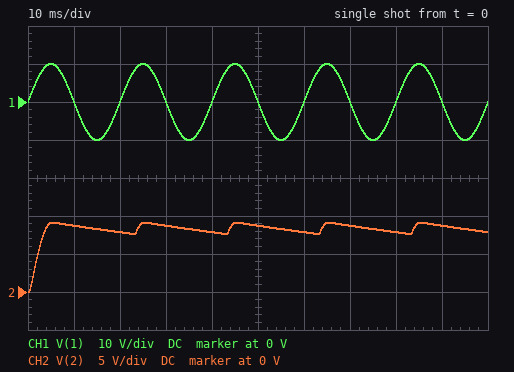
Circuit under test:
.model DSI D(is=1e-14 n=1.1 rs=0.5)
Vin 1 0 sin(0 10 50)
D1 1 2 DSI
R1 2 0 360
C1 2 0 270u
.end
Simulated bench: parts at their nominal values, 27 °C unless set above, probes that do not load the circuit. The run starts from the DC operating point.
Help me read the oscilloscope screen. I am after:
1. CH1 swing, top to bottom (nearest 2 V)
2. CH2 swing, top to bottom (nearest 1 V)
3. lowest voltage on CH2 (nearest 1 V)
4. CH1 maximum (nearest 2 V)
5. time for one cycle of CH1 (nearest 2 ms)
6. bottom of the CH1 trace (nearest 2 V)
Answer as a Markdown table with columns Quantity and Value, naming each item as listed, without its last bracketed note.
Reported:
| Quantity | Value |
|---|---|
| CH1 swing, top to bottom | 20 V |
| CH2 swing, top to bottom | 9 V |
| lowest voltage on CH2 | 0 V |
| CH1 maximum | 10 V |
| time for one cycle of CH1 | 20 ms |
| bottom of the CH1 trace | -10 V |
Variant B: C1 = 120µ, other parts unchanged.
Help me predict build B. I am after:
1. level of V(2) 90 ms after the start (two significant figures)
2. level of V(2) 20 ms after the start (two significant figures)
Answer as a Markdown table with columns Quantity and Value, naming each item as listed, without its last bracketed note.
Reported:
| Quantity | Value |
|---|---|
| level of V(2) 90 ms after the start | 8.2 V |
| level of V(2) 20 ms after the start | 6.5 V |
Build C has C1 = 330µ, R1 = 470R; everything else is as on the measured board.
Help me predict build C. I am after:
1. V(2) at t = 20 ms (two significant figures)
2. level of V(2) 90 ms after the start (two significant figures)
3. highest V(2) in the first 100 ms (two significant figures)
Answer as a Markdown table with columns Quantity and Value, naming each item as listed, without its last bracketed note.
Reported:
| Quantity | Value |
|---|---|
| V(2) at t = 20 ms | 8.3 V |
| level of V(2) 90 ms after the start | 8.9 V |
| highest V(2) in the first 100 ms | 9.1 V |
